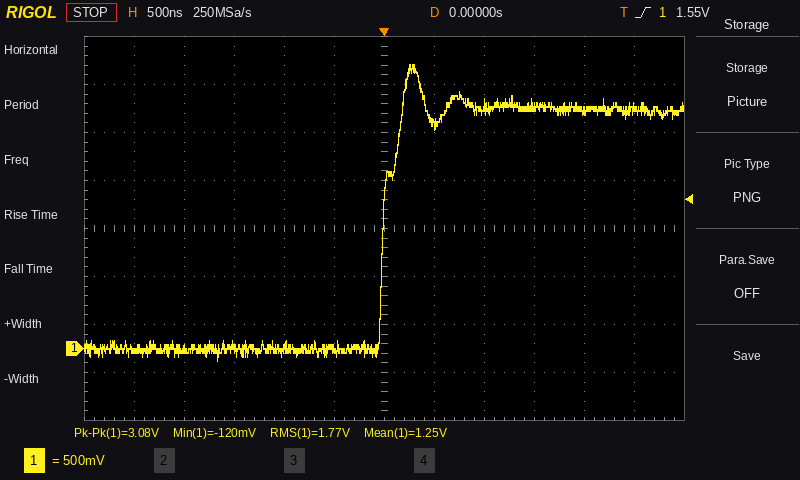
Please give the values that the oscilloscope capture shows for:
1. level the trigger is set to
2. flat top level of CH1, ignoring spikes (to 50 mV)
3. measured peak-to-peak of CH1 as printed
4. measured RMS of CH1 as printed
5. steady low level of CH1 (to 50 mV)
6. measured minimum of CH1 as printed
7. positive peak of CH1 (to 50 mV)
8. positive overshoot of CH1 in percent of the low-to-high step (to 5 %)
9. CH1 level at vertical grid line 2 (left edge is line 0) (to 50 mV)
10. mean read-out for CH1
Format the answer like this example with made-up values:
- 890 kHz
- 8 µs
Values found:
- 1.55 V
- 2.50 V
- 3.08 V
- 1.77 V
- 0 mV
- -120 mV
- 2.95 V
- 20 %
- 0 mV
- 1.25 V
